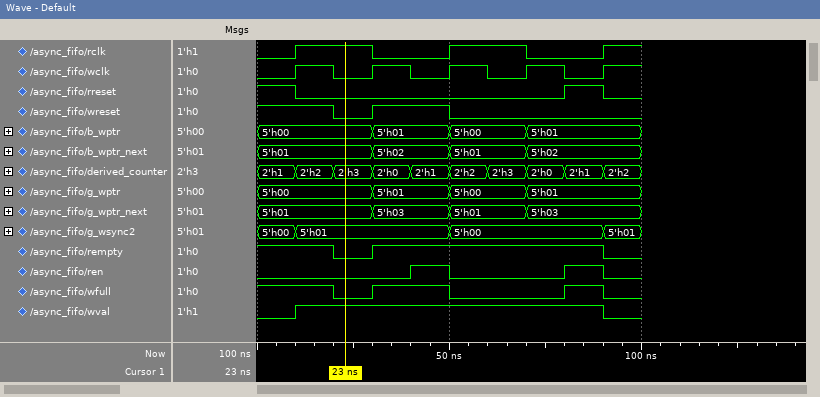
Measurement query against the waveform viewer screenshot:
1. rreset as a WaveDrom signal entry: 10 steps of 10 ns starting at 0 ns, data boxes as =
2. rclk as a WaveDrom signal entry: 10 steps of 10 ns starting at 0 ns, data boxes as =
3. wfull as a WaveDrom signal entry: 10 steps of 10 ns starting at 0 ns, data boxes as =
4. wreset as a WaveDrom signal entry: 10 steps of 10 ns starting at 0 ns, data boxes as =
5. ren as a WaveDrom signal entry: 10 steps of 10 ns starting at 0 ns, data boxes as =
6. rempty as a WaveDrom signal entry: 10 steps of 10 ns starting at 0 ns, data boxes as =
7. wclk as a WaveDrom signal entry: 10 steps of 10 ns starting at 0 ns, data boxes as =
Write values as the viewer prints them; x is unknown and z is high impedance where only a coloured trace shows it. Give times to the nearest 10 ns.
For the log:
{name: 'rreset', wave: '10......10'}
{name: 'rclk', wave: '01.0.1.0.1'}
{name: 'wfull', wave: '1.01.0..10'}
{name: 'wreset', wave: '1.01.0....'}
{name: 'ren', wave: '0...10..10'}
{name: 'rempty', wave: '1.01.....0'}
{name: 'wclk', wave: '0101010101'}
